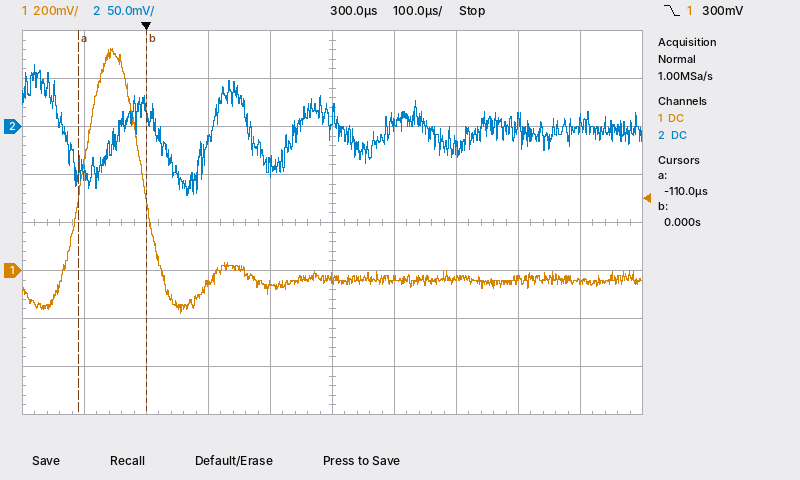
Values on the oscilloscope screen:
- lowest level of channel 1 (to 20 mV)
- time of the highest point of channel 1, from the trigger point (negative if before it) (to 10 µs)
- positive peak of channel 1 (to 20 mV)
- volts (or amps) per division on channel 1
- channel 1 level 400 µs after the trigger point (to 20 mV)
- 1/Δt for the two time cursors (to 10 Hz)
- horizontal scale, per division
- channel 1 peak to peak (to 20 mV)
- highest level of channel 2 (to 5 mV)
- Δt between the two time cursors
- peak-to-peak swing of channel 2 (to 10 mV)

-180 mV
-60 µs
920 mV
200 mV
-40 mV
9.09 kHz
100 µs
1.10 V
65 mV
110 µs
140 mV
